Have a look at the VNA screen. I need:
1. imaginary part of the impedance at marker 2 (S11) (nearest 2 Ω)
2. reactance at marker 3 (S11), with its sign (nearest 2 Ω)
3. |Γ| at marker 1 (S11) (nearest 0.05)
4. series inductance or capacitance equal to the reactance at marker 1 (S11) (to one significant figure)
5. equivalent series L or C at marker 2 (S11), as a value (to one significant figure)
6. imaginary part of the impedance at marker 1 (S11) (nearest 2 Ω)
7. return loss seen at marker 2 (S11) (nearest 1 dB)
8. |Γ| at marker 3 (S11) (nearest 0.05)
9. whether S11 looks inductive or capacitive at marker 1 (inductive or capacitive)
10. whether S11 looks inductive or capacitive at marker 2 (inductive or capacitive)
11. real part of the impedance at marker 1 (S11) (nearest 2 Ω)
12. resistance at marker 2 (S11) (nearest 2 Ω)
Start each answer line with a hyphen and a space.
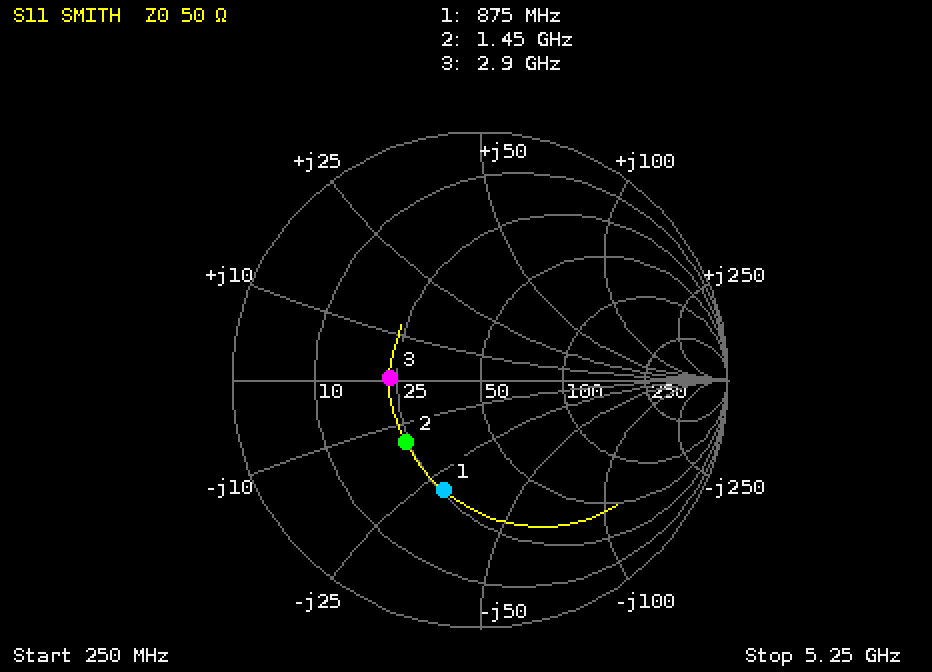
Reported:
- -14 Ω
- 0 Ω
- 0.45
- 6 pF
- 8 pF
- -30 Ω
- 8 dB
- 0.35
- capacitive
- capacitive
- 26 Ω
- 24 Ω
